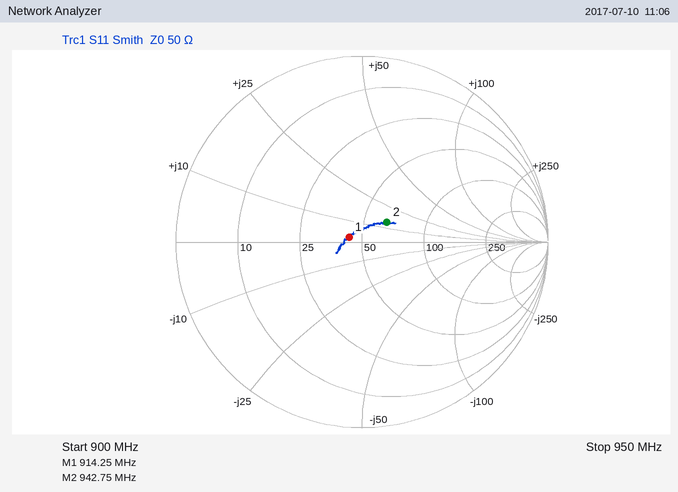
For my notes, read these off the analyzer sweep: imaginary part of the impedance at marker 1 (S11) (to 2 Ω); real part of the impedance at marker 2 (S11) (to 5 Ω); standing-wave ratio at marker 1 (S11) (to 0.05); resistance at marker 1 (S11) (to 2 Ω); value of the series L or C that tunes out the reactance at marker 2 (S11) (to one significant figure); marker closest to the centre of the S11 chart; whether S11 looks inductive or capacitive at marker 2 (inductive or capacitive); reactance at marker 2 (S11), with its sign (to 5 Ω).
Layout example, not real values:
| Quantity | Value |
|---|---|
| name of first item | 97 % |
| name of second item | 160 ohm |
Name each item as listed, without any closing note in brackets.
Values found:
| Quantity | Value |
|---|---|
| imaginary part of the impedance at marker 1 (S11) | +2 Ω |
| real part of the impedance at marker 2 (S11) | 65 Ω |
| standing-wave ratio at marker 1 (S11) | 1.15 |
| resistance at marker 1 (S11) | 44 Ω |
| value of the series L or C that tunes out the reactance at marker 2 (S11) | 10 pF |
| marker closest to the centre of the S11 chart | marker 1 |
| whether S11 looks inductive or capacitive at marker 2 | inductive |
| reactance at marker 2 (S11), with its sign | +15 Ω |
